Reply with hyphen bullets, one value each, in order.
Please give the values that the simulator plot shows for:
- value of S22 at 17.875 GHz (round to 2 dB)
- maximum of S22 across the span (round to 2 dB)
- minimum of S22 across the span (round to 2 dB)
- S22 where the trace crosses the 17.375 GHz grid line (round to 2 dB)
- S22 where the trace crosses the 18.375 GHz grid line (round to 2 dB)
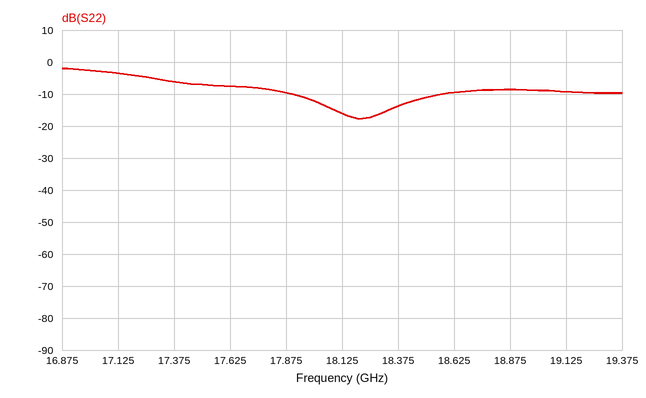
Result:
- -10 dB
- -2 dB
- -18 dB
- -6 dB
- -14 dB
